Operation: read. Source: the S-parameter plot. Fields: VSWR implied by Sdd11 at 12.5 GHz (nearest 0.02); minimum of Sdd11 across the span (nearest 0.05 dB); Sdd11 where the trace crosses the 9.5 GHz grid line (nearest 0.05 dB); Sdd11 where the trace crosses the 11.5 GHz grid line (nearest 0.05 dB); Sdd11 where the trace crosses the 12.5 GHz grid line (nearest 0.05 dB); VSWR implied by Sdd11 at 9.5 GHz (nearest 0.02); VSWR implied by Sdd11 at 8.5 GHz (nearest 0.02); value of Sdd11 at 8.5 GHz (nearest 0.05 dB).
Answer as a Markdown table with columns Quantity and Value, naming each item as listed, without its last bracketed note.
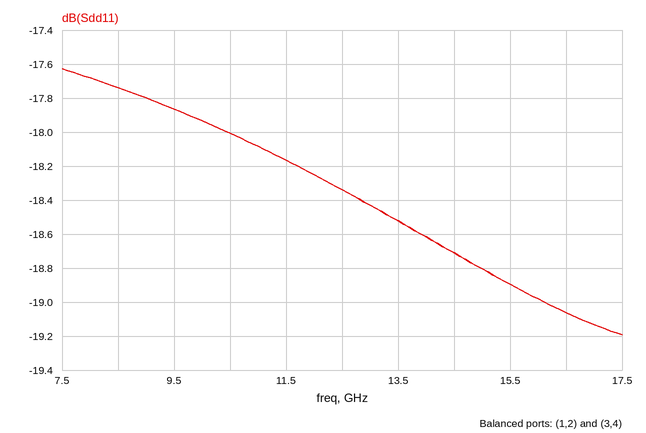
| Quantity | Value |
|---|---|
| VSWR implied by Sdd11 at 12.5 GHz | 1.28 |
| minimum of Sdd11 across the span | -19.20 dB |
| Sdd11 where the trace crosses the 9.5 GHz grid line | -17.85 dB |
| Sdd11 where the trace crosses the 11.5 GHz grid line | -18.15 dB |
| Sdd11 where the trace crosses the 12.5 GHz grid line | -18.35 dB |
| VSWR implied by Sdd11 at 9.5 GHz | 1.30 |
| VSWR implied by Sdd11 at 8.5 GHz | 1.30 |
| value of Sdd11 at 8.5 GHz | -17.75 dB |
